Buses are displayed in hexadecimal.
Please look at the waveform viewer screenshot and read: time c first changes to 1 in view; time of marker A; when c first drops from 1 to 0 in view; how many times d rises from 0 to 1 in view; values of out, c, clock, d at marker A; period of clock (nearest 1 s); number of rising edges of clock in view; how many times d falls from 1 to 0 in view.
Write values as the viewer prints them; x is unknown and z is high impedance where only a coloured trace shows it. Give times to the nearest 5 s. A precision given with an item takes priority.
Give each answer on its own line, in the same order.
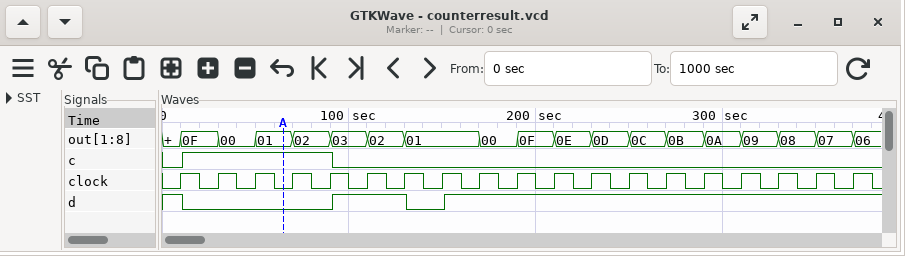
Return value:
10 s
65 s
90 s
2
out=01, c=1, clock=0, d=0
20 s
19
2
